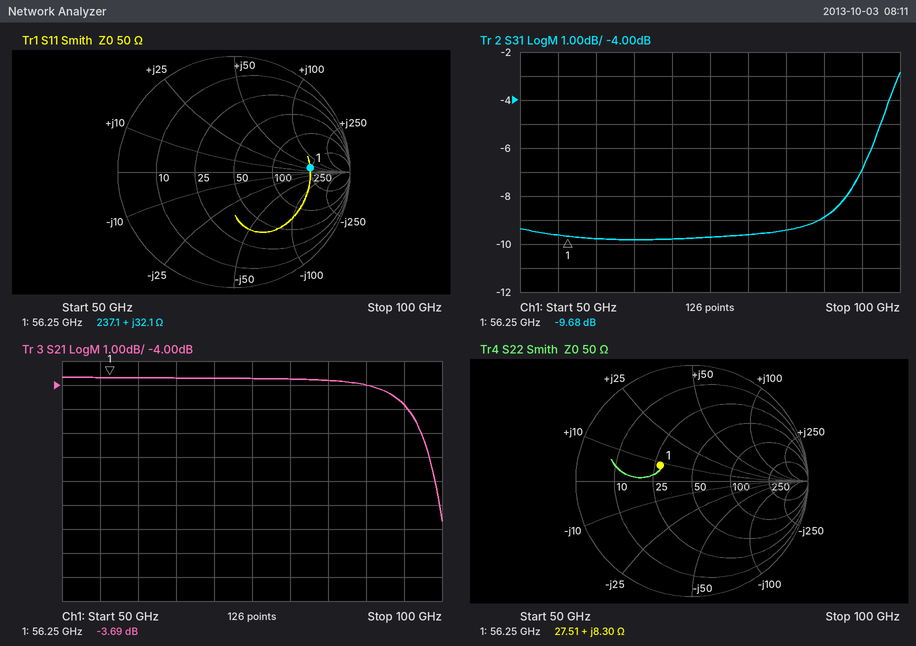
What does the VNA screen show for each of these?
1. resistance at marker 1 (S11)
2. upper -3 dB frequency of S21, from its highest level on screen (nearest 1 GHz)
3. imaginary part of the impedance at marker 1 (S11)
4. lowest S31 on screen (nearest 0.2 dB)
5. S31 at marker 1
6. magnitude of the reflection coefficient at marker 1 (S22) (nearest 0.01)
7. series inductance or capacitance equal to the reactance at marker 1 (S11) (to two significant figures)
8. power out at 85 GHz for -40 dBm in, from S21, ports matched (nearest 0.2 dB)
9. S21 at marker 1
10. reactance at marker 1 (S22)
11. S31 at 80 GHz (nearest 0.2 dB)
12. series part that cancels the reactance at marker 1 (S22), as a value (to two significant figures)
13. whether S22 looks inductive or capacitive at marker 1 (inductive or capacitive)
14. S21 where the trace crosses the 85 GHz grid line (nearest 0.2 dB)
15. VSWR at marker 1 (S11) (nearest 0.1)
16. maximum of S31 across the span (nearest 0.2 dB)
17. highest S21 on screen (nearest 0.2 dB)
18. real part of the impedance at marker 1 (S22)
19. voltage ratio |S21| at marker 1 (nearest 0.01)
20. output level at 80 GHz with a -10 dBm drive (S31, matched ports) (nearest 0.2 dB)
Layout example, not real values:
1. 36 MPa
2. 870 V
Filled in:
1. 237.1 Ω
2. 98 GHz
3. +32.1 Ω
4. -9.8 dB
5. -9.68 dB
6. 0.31
7. 91 pH
8. -43.8 dBm
9. -3.69 dB
10. +8.30 Ω
11. -9.6 dB
12. 340 fF
13. inductive
14. -3.8 dB
15. 4.8
16. -2.8 dB
17. -3.6 dB
18. 27.51 Ω
19. 0.65
20. -19.6 dBm
